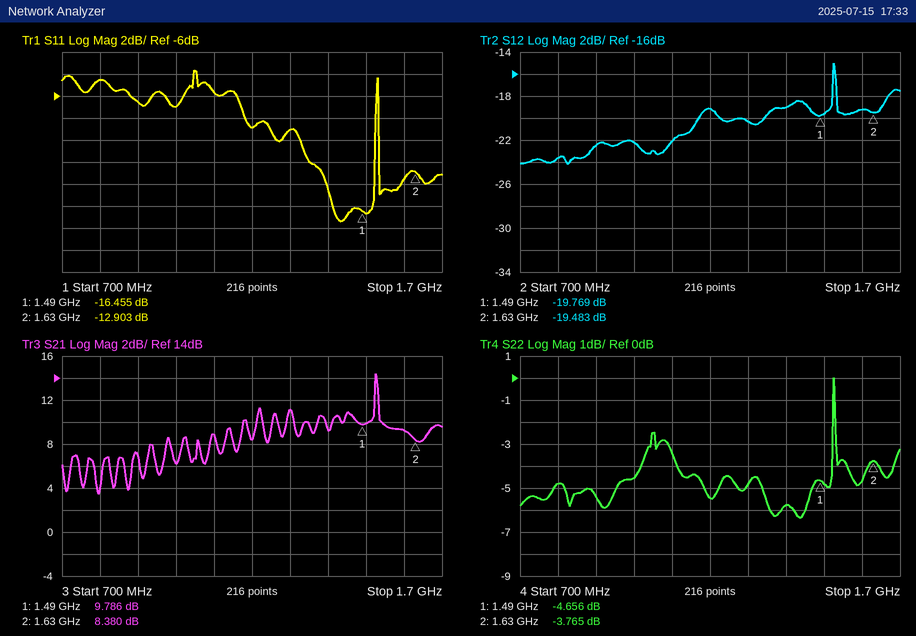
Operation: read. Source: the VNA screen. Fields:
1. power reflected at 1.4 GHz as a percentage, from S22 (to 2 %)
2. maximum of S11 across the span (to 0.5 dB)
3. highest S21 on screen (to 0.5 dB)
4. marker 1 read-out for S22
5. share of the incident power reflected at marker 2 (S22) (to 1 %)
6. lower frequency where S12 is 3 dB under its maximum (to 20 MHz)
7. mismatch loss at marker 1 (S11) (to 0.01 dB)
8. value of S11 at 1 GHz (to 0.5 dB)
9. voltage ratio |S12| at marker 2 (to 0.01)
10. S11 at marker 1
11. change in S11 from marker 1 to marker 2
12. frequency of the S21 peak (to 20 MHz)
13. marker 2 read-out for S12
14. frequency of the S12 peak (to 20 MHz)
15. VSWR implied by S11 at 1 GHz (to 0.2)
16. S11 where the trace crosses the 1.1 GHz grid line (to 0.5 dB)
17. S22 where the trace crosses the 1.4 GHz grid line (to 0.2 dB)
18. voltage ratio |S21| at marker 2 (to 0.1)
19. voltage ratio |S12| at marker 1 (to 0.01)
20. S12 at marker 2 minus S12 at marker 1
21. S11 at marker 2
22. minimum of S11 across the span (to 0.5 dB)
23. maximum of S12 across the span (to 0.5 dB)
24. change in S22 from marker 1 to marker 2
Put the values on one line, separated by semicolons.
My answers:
26 %; -3.5 dB; 14.5 dB; -4.656 dB; 42 %; 1.52 GHz; 0.10 dB; -7.0 dB; 0.11; -16.455 dB; 3.552 dB; 1.52 GHz; -19.483 dB; 1.52 GHz; 2.6; -5.5 dB; -5.8 dB; 2.6; 0.10; 0.286 dB; -12.903 dB; -17.5 dB; -15.0 dB; 0.891 dB
